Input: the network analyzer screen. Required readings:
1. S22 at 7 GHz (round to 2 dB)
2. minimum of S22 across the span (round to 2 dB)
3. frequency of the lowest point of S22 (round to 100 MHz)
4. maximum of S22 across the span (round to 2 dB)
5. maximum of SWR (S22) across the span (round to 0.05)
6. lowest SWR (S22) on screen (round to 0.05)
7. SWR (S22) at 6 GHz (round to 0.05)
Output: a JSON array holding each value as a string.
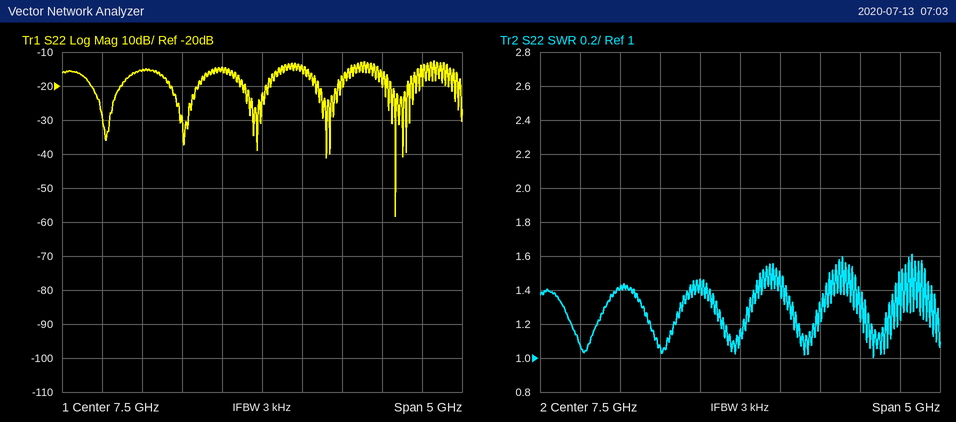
["-14 dB", "-58 dB", "9.2 GHz", "-12 dB", "1.60", "1.00", "1.40"]
